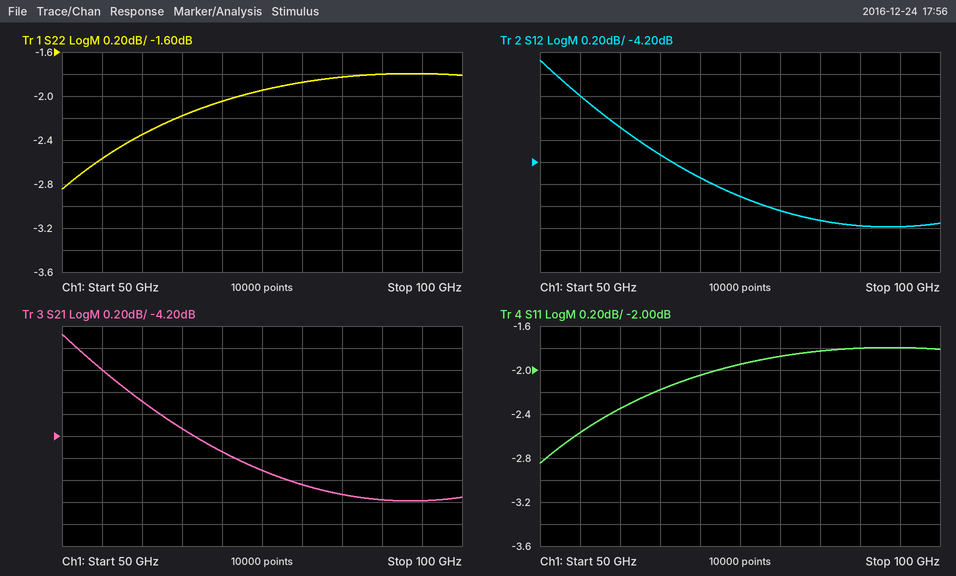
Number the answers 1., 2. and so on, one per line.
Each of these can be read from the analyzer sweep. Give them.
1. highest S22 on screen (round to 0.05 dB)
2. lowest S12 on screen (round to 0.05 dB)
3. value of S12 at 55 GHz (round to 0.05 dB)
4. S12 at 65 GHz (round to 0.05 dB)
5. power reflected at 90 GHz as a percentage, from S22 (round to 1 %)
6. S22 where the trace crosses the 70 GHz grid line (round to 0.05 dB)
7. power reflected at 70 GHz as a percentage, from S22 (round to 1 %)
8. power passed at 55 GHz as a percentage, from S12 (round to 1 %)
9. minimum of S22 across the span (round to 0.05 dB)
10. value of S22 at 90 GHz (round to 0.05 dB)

1. -1.80 dB
2. -4.80 dB
3. -3.60 dB
4. -4.15 dB
5. 66 %
6. -2.05 dB
7. 62 %
8. 44 %
9. -2.85 dB
10. -1.80 dB
